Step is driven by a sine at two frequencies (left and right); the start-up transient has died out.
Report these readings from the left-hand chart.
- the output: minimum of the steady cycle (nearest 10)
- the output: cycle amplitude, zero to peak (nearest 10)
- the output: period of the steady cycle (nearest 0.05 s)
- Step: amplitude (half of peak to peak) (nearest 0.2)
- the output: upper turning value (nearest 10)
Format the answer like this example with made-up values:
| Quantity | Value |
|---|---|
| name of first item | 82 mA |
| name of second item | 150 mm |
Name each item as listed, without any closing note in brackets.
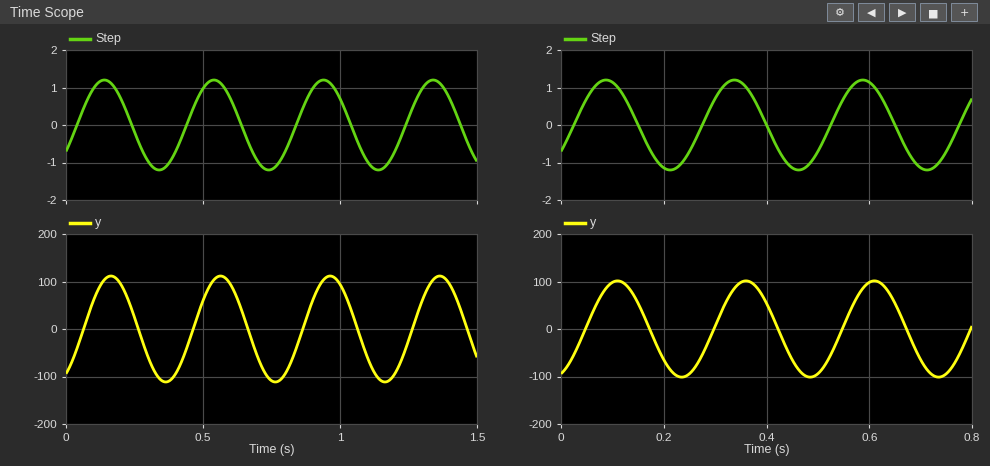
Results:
| Quantity | Value |
|---|---|
| the output: minimum of the steady cycle | -110 |
| the output: cycle amplitude, zero to peak | 110 |
| the output: period of the steady cycle | 0.40 s |
| Step: amplitude (half of peak to peak) | 1.2 |
| the output: upper turning value | 110 |
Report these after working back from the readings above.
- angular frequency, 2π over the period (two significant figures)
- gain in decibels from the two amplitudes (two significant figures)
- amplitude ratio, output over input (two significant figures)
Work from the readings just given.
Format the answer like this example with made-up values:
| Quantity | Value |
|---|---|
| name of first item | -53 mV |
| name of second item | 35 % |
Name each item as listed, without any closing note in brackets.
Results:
| Quantity | Value |
|---|---|
| angular frequency, 2π over the period | 16 rad/s |
| gain in decibels from the two amplitudes | 39 dB |
| amplitude ratio, output over input | 92 |
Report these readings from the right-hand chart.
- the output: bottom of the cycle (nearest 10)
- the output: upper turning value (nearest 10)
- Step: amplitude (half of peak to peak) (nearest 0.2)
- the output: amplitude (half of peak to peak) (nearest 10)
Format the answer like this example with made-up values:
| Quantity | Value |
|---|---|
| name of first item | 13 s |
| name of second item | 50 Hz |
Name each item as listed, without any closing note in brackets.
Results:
| Quantity | Value |
|---|---|
| the output: bottom of the cycle | -100 |
| the output: upper turning value | 100 |
| Step: amplitude (half of peak to peak) | 1.2 |
| the output: amplitude (half of peak to peak) | 100 |
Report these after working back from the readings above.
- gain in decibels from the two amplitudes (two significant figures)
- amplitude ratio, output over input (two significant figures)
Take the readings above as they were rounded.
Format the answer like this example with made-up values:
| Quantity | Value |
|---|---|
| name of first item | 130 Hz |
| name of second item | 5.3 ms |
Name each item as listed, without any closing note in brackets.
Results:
| Quantity | Value |
|---|---|
| gain in decibels from the two amplitudes | 38 dB |
| amplitude ratio, output over input | 83 |
